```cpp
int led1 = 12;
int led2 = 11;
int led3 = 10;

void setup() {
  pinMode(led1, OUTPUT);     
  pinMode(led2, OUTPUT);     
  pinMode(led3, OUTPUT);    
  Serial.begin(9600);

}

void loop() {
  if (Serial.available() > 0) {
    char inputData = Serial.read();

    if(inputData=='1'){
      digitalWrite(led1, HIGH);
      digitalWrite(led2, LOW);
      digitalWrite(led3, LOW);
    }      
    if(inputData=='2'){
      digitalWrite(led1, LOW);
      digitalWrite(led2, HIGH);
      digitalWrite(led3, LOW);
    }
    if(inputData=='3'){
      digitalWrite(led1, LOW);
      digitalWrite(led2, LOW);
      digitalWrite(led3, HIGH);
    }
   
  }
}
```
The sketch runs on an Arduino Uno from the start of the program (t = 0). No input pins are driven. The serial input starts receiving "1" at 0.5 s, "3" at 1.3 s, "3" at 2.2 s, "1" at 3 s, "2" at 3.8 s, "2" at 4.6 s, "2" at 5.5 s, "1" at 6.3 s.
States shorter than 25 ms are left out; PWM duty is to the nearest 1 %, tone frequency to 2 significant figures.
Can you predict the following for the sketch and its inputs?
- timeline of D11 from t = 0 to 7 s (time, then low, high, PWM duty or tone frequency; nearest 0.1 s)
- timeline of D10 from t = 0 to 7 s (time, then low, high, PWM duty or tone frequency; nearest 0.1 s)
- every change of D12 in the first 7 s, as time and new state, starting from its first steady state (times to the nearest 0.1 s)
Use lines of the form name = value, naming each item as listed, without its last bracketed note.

timeline of D11 from t = 0 to 7 s = 0 s low; 3.8 s high; 6.3 s low
timeline of D10 from t = 0 to 7 s = 0 s low; 1.3 s high; 3 s low
every change of D12 in the first 7 s, as time and new state, starting from its first steady state = 0 s low; 0.5 s high; 1.3 s low; 3 s high; 3.8 s low; 6.3 s high
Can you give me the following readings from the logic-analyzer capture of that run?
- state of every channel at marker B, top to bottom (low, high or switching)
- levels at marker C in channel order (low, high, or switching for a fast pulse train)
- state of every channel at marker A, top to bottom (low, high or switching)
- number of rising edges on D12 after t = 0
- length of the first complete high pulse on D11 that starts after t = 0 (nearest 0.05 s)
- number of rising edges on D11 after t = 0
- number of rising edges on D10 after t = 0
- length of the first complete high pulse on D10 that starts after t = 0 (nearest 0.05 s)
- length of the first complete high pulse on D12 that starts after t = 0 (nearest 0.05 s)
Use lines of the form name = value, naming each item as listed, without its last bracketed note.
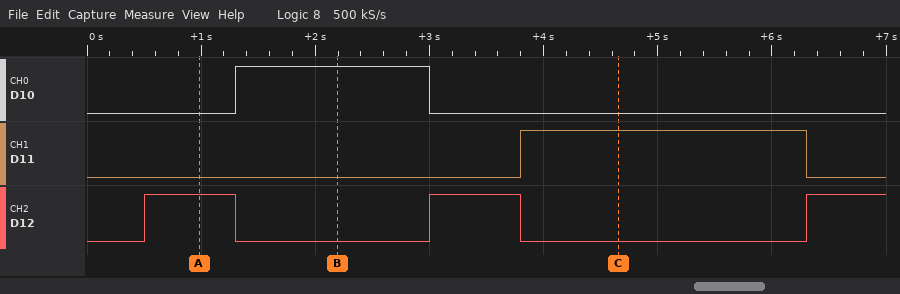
state of every channel at marker B, top to bottom = D10 high, D11 low, D12 low
levels at marker C in channel order = D10 low, D11 high, D12 low
state of every channel at marker A, top to bottom = D10 low, D11 low, D12 high
number of rising edges on D12 after t = 0 = 3
length of the first complete high pulse on D11 that starts after t = 0 = 2.50 s
number of rising edges on D11 after t = 0 = 1
number of rising edges on D10 after t = 0 = 1
length of the first complete high pulse on D10 that starts after t = 0 = 1.70 s
length of the first complete high pulse on D12 that starts after t = 0 = 0.80 s
